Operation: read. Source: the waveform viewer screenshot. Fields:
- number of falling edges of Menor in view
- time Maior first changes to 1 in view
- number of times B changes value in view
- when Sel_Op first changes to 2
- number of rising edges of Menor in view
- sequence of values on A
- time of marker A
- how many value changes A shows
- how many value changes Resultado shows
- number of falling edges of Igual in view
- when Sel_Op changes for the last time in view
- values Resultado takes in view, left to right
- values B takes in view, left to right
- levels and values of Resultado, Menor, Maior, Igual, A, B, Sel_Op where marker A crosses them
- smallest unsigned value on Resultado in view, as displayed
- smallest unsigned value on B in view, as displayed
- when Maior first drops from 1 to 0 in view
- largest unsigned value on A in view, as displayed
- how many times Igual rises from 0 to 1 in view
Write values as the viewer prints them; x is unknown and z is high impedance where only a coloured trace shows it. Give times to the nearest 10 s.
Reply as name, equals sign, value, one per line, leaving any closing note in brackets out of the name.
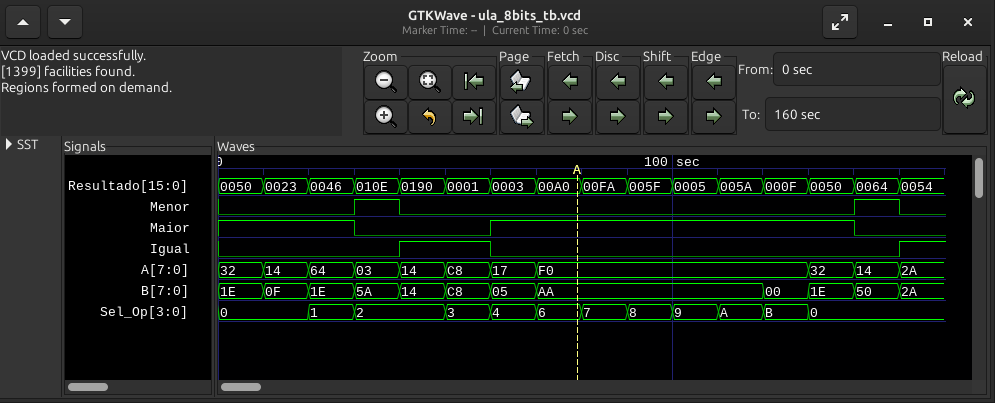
number of falling edges of Menor in view = 2
time Maior first changes to 1 in view = 60 s
number of times B changes value in view = 11
when Sel_Op first changes to 2 = 30 s
number of rising edges of Menor in view = 2
sequence of values on A = 32, 14, 64, 03, 14, C8, 17, F0, 32, 14, 2A
time of marker A = 80 s
how many value changes A shows = 10
how many value changes Resultado shows = 15
number of falling edges of Igual in view = 1
when Sel_Op changes for the last time in view = 130 s
values Resultado takes in view, left to right = 0050, 0023, 0046, 010E, 0190, 0001, 0003, 00A0, 00FA, 005F, 0005, 005A, 000F, 0050, 0064, 0054
values B takes in view, left to right = 1E, 0F, 1E, 5A, 14, C8, 05, AA, 00, 1E, 50, 2A
levels and values of Resultado, Menor, Maior, Igual, A, B, Sel_Op where marker A crosses them = Resultado=00A0, Menor=0, Maior=1, Igual=0, A=F0, B=AA, Sel_Op=6
smallest unsigned value on Resultado in view, as displayed = 0001
smallest unsigned value on B in view, as displayed = 00
when Maior first drops from 1 to 0 in view = 30 s
largest unsigned value on A in view, as displayed = F0
how many times Igual rises from 0 to 1 in view = 2
